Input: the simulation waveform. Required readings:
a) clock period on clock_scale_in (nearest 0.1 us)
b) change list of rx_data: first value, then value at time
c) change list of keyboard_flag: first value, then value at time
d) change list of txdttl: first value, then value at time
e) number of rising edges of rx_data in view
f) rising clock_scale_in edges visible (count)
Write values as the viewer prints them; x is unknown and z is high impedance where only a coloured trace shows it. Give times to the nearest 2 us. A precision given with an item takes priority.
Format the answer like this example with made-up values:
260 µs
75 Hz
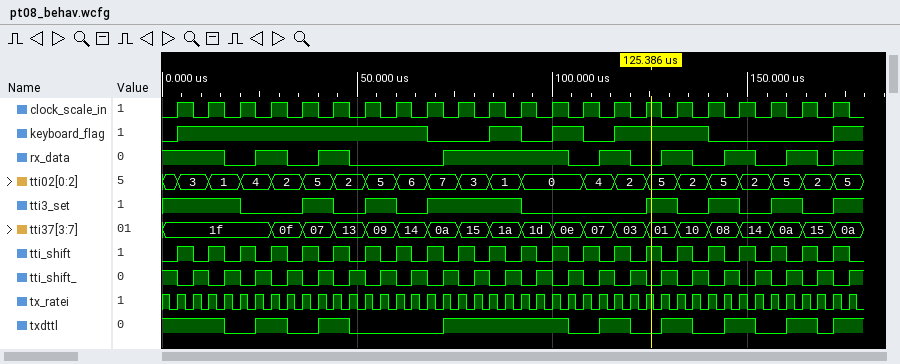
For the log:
8 us
1, 0 at 16 us, 1 at 24 us, 0 at 32 us, 1 at 40 us, 0 at 48 us, 1 at 72 us, 0 at 104 us, 1 at 112 us, 0 at 120 us, 1 at 128 us, 0 at 136 us, 1 at 144 us, 0 at 152 us, 1 at 160 us, 0 at 168 us, 1 at 172 us
0, 1 at 4 us, 0 at 68 us, 1 at 84 us, 0 at 92 us, 1 at 100 us, 0 at 108 us, 1 at 116 us, 0 at 140 us, 1 at 172 us
1, 0 at 16 us, 1 at 24 us, 0 at 32 us, 1 at 40 us, 0 at 48 us, 1 at 72 us, 0 at 104 us, 1 at 112 us, 0 at 120 us, 1 at 128 us, 0 at 136 us, 1 at 144 us, 0 at 152 us, 1 at 160 us, 0 at 168 us, 1 at 172 us
8
22
